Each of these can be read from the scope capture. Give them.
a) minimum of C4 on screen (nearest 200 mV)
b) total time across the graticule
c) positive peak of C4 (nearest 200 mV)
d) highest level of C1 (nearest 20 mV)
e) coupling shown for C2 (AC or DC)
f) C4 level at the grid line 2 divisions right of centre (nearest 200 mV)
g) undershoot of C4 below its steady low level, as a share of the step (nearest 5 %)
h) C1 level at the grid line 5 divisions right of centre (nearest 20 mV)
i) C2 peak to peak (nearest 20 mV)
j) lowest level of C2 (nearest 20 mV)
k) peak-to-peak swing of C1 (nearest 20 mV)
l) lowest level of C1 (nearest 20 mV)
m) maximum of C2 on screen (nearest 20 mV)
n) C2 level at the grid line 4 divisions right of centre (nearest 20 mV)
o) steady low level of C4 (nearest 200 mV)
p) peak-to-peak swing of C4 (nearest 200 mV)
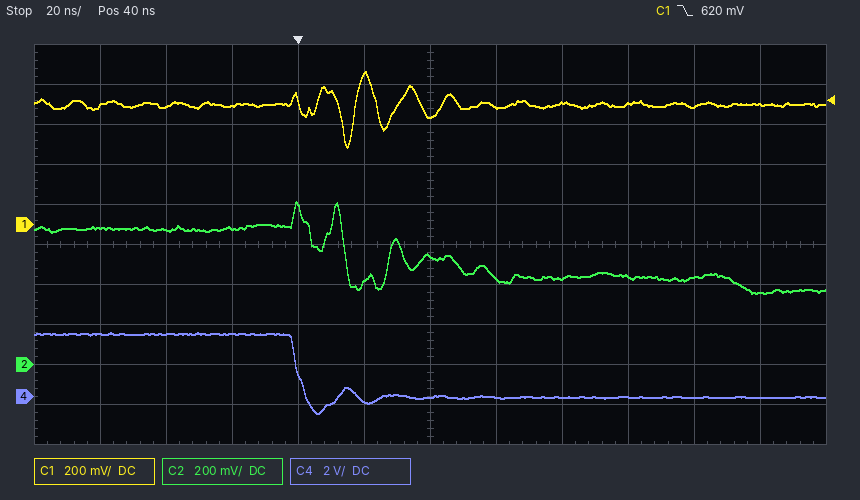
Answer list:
-800 mV
240 ns
3.2 V
760 mV
DC
0.0 V
25 %
600 mV
460 mV
360 mV
380 mV
380 mV
820 mV
440 mV
0.0 V
4.0 V
